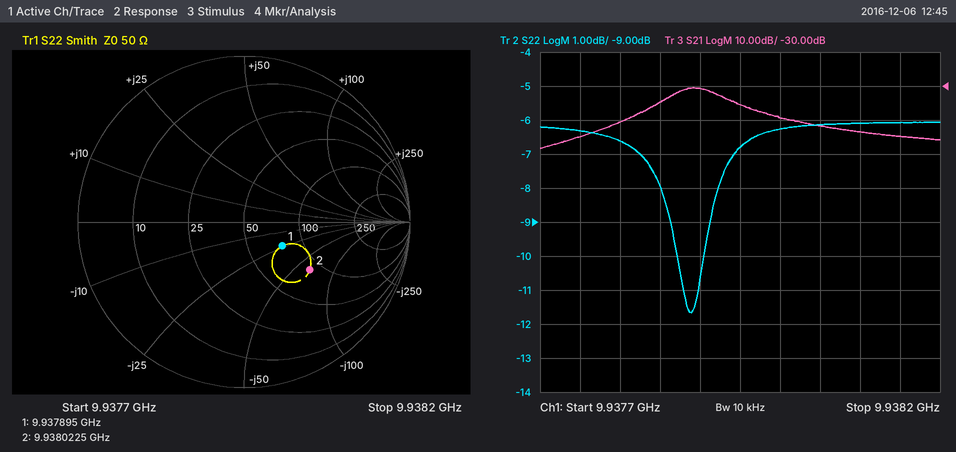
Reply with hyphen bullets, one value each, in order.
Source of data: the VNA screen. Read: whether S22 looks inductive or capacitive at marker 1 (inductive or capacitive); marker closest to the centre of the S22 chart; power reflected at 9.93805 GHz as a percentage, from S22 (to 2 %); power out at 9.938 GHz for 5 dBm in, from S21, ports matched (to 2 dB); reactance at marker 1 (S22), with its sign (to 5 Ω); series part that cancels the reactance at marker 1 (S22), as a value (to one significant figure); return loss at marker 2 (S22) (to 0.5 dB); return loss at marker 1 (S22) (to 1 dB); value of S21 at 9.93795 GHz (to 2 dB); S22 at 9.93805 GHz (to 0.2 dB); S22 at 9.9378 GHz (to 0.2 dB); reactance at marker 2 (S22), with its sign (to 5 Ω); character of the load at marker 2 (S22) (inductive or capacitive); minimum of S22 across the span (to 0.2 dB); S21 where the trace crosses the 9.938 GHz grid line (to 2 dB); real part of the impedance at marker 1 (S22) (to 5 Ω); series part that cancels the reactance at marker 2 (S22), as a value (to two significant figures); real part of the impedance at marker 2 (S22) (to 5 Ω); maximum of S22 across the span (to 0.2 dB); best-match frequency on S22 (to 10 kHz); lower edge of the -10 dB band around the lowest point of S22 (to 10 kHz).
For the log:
- capacitive
- marker 1
- 24 %
- -34 dBm
- -25 Ω
- 400 pH
- 6.0 dB
- 11 dB
- -36 dB
- -6.2 dB
- -6.6 dB
- -65 Ω
- capacitive
- -11.6 dB
- -40 dB
- 75 Ω
- 1.0 nH
- 85 Ω
- -6.0 dB
- 9.93789 GHz
- 9.93787 GHz
